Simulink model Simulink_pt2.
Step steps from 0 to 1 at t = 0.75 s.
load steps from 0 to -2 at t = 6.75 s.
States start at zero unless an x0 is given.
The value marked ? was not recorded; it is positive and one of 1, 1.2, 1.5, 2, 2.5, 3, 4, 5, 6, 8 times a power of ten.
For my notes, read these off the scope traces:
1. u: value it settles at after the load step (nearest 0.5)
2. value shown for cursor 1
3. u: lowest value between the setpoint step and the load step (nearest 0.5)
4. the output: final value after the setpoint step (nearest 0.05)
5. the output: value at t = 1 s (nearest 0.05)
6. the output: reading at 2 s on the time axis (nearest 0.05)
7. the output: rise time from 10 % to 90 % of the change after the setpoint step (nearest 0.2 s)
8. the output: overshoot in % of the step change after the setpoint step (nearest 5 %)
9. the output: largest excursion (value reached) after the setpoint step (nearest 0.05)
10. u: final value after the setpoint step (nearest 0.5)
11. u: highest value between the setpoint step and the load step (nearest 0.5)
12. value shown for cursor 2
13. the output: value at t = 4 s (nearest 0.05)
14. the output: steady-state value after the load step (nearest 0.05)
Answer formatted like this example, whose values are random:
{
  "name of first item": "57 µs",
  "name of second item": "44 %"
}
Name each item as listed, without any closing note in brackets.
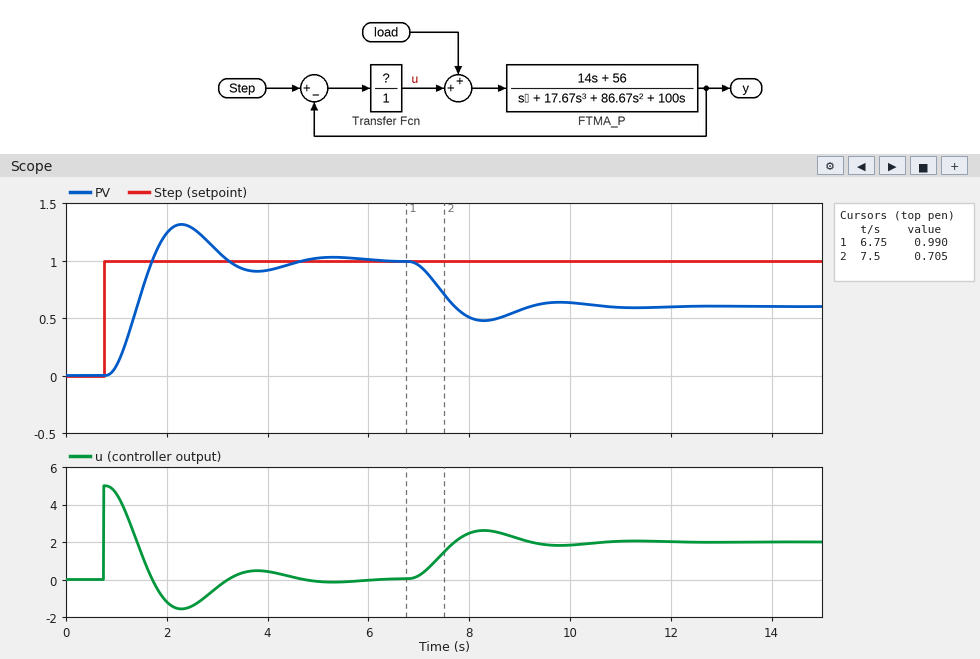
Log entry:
{
  "u: value it settles at after the load step": "2.0",
  "value shown for cursor 1": "0.990",
  "u: lowest value between the setpoint step and the load step": "-1.5",
  "the output: final value after the setpoint step": "1.00",
  "the output: value at t = 1 s": "0.10",
  "the output: reading at 2 s on the time axis": "1.25",
  "the output: rise time from 10 % to 90 % of the change after the setpoint step": "0.6 s",
  "the output: overshoot in % of the step change after the setpoint step": "30 %",
  "the output: largest excursion (value reached) after the setpoint step": "1.30",
  "u: final value after the setpoint step": "0.0",
  "u: highest value between the setpoint step and the load step": "5.0",
  "value shown for cursor 2": "0.705",
  "the output: value at t = 4 s": "0.90",
  "the output: steady-state value after the load step": "0.60"
}
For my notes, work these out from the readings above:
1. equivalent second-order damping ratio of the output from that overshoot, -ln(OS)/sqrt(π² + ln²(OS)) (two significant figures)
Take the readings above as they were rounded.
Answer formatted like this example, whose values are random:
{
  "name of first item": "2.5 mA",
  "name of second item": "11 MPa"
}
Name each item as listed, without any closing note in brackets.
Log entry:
{
  "equivalent second-order damping ratio of the output from that overshoot, -ln(OS)/sqrt(π² + ln²(OS))": "0.36"
}
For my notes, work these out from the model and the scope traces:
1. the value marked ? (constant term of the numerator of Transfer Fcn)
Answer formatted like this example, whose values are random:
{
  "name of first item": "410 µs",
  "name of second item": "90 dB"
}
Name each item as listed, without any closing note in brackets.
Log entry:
{
  "the value marked ?": "5"
}
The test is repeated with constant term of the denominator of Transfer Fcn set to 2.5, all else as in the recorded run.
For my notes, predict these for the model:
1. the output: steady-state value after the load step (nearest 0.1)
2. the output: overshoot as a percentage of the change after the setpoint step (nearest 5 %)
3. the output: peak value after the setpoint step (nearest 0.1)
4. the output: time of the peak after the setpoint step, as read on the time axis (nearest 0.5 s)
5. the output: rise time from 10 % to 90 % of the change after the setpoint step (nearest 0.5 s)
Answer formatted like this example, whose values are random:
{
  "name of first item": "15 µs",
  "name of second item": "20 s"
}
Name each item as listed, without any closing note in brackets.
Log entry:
{
  "the output: steady-state value after the load step": "0.0",
  "the output: overshoot as a percentage of the change after the setpoint step": "10 %",
  "the output: peak value after the setpoint step": "1.1",
  "the output: time of the peak after the setpoint step, as read on the time axis": "3.5 s",
  "the output: rise time from 10 % to 90 % of the change after the setpoint step": "1.5 s"
}
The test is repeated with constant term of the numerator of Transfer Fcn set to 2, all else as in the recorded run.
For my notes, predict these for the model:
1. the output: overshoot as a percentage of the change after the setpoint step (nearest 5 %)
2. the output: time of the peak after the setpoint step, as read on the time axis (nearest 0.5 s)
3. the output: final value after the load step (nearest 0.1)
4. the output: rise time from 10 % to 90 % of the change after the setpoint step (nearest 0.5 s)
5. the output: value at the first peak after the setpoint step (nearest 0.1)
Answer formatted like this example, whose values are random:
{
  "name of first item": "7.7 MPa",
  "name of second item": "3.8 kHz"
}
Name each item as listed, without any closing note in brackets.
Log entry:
{
  "the output: overshoot as a percentage of the change after the setpoint step": "10 %",
  "the output: time of the peak after the setpoint step, as read on the time axis": "3.5 s",
  "the output: final value after the load step": "0.0",
  "the output: rise time from 10 % to 90 % of the change after the setpoint step": "1.5 s",
  "the output: value at the first peak after the setpoint step": "1.1"
}
